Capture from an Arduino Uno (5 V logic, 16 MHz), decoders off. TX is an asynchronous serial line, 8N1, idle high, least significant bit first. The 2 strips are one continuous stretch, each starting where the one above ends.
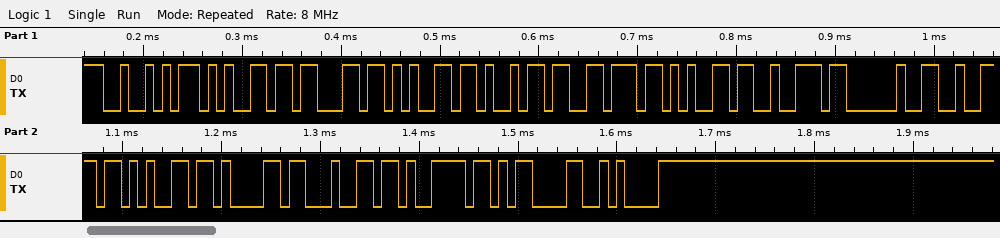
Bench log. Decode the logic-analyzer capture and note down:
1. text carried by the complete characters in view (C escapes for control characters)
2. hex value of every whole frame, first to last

"Receiver ready\r\n"
52 65 63 65 69 76 65 72 20 72 65 61 64 79 0D 0A
